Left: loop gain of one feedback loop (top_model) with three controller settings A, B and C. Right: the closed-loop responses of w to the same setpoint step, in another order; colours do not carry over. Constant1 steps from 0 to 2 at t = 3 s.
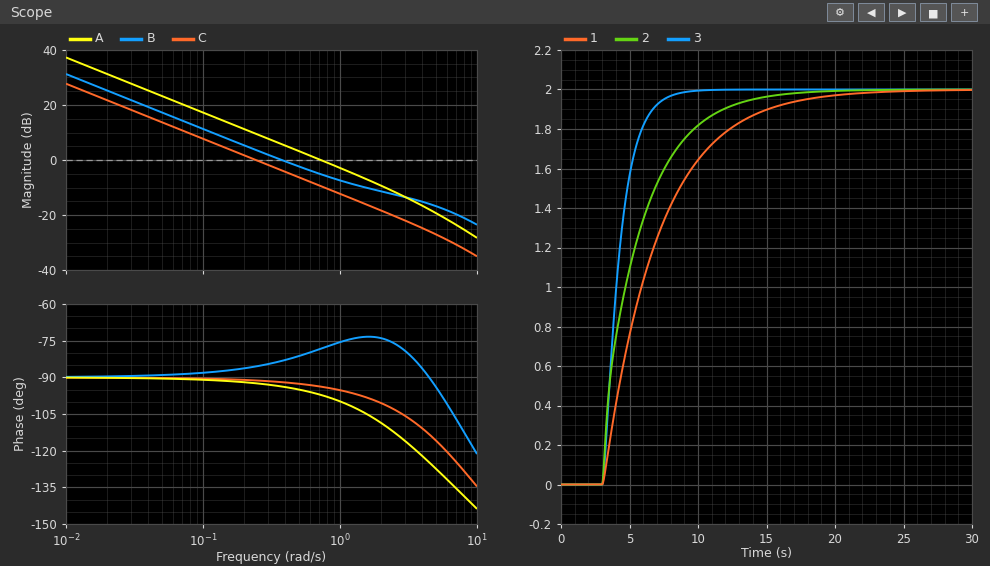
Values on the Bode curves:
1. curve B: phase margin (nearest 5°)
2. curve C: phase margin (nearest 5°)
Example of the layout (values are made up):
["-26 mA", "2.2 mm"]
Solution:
["95°", "90°"]
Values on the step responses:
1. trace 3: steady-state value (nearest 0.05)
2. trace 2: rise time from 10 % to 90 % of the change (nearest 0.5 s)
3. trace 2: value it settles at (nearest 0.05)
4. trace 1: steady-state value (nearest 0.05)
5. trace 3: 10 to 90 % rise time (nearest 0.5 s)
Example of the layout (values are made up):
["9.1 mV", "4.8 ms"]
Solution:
["2.00", "6.5 s", "2.00", "2.00", "2.5 s"]
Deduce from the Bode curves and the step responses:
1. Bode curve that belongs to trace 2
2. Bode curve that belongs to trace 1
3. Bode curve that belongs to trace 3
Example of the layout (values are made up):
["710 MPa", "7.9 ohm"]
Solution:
["B", "C", "A"]
